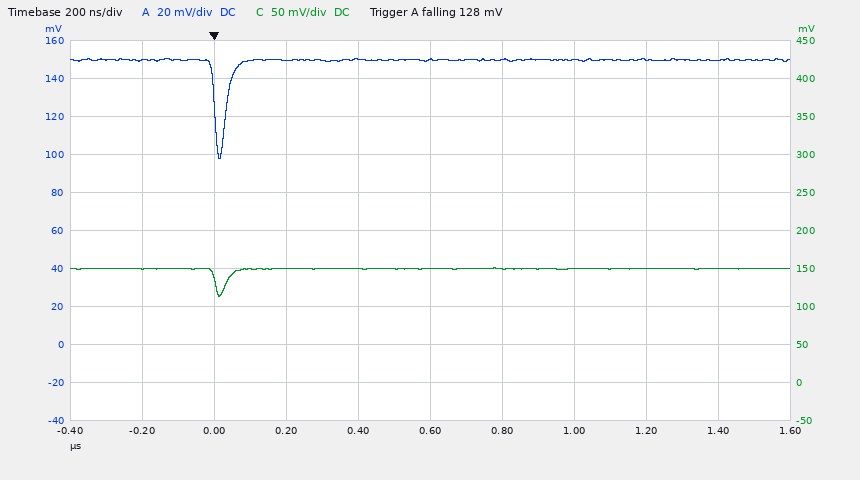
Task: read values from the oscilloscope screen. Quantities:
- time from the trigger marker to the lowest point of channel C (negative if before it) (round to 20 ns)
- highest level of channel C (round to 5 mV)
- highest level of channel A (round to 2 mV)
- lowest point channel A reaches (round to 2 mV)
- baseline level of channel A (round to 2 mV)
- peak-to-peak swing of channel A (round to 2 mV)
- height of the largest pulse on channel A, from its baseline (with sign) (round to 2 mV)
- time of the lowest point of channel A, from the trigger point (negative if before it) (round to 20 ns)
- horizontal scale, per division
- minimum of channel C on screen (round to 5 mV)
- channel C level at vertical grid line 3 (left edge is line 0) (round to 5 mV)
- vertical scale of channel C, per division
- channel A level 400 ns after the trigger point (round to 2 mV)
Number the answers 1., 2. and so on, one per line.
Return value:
1. +20 ns
2. 150 mV
3. 150 mV
4. 98 mV
5. 150 mV
6. 52 mV
7. -52 mV
8. +20 ns
9. 200 ns
10. 115 mV
11. 150 mV
12. 50 mV
13. 150 mV
